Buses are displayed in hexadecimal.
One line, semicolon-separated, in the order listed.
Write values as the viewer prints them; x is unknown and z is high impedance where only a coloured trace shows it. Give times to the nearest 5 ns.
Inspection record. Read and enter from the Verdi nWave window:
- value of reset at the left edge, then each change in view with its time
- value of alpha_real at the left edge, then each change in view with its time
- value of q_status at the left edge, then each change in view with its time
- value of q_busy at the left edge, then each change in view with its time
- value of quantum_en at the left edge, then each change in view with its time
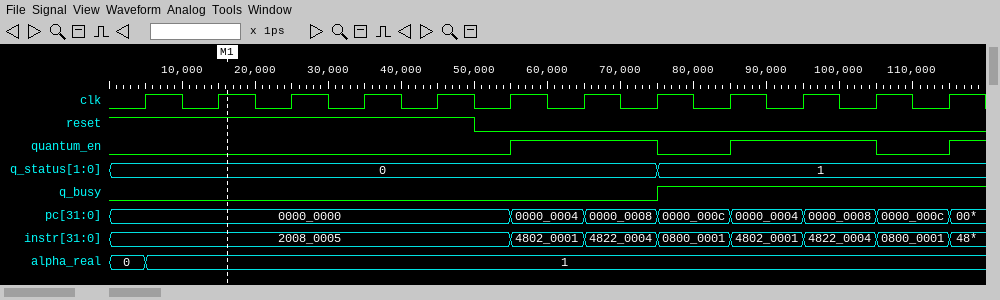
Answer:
1, 0 at 50 ns; 0, 1 at 5 ns; 0, 1 at 75 ns; 0, 1 at 75 ns; 0, 1 at 55 ns, 0 at 75 ns, 1 at 85 ns, 0 at 105 ns, 1 at 115 ns
